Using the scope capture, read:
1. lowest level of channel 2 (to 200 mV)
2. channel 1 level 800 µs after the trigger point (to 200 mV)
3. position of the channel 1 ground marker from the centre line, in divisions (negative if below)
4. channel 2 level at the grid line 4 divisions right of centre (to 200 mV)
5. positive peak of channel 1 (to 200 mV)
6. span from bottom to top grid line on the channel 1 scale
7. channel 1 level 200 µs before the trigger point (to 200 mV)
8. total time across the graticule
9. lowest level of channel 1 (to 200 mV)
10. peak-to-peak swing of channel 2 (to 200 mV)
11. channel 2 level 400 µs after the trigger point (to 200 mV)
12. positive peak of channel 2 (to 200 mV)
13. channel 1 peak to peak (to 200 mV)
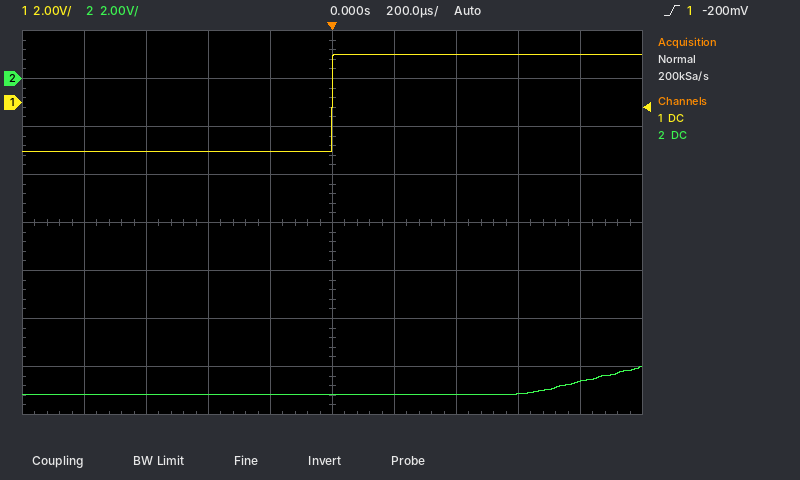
-13.2 V
2.0 V
+2.5 div
-12.6 V
2.0 V
16 V
-2.0 V
2 ms
-2.0 V
1.2 V
-13.2 V
-12.0 V
4.0 V
